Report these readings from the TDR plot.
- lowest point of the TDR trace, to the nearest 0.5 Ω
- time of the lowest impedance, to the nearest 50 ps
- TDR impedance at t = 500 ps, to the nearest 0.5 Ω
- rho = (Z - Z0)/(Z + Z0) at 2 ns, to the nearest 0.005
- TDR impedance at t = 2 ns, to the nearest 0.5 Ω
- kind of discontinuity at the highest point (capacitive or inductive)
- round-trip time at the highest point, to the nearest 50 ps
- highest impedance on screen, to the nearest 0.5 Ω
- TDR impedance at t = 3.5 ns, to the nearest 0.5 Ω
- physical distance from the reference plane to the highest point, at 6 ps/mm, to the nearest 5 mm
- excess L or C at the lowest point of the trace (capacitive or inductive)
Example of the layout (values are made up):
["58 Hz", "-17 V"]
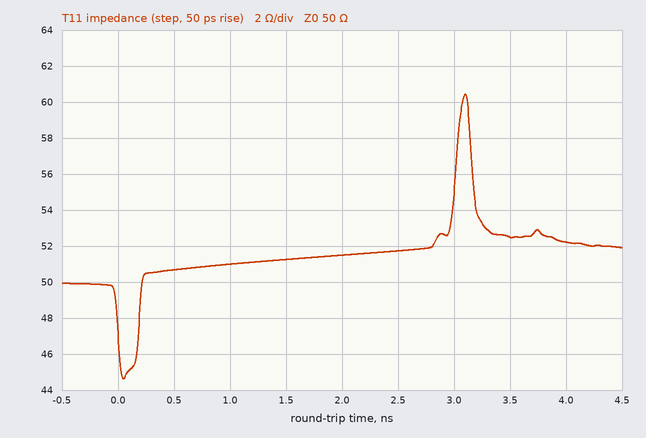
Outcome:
["44.5 Ω", "50 ps", "50.5 Ω", "+0.015", "51.5 Ω", "inductive", "3.10 ns", "60.5 Ω", "52.5 Ω", "260 mm", "capacitive"]
